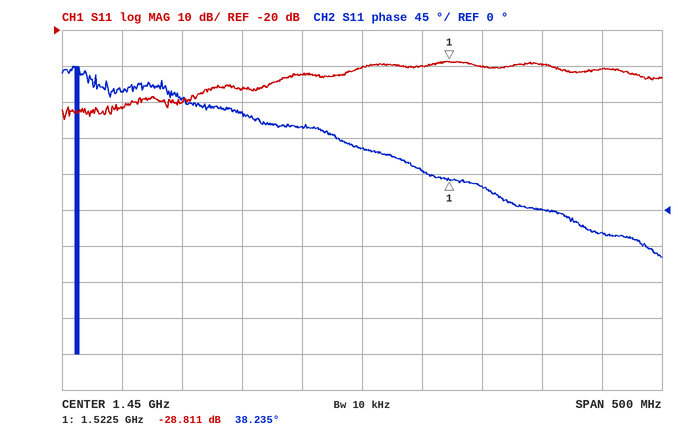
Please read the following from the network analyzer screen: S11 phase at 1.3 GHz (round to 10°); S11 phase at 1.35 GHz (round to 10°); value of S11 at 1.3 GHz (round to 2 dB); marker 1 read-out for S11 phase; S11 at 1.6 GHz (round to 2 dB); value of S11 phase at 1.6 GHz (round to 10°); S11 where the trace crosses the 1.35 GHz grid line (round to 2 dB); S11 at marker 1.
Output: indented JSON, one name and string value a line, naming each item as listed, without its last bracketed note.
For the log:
{
  "S11 phase at 1.3 GHz": "140°",
  "S11 phase at 1.35 GHz": "120°",
  "value of S11 at 1.3 GHz": "-40 dB",
  "marker 1 read-out for S11 phase": "38.235°",
  "S11 at 1.6 GHz": "-30 dB",
  "value of S11 phase at 1.6 GHz": "0°",
  "S11 where the trace crosses the 1.35 GHz grid line": "-36 dB",
  "S11 at marker 1": "-28.811 dB"
}
